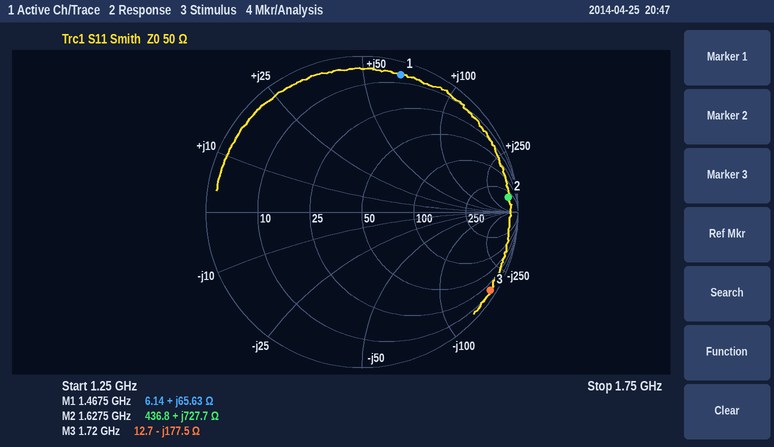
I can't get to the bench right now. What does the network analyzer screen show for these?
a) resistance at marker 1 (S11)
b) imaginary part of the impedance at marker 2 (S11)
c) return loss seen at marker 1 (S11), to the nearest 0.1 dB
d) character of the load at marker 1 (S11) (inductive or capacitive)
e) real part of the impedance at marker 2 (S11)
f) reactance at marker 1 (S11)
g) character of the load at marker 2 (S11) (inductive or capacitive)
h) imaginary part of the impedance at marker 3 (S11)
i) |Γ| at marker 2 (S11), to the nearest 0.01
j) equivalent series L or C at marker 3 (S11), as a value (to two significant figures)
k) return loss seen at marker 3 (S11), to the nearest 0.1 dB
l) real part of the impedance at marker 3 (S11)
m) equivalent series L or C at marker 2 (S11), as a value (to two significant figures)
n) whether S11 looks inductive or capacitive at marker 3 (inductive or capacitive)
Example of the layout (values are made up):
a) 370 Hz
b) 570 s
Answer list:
a) 6.14 Ω
b) +727.7 Ω
c) 0.8 dB
d) inductive
e) 436.8 Ω
f) +65.63 Ω
g) inductive
h) -177.5 Ω
i) 0.94
j) 520 fF
k) 0.3 dB
l) 12.7 Ω
m) 71 nH
n) capacitive
